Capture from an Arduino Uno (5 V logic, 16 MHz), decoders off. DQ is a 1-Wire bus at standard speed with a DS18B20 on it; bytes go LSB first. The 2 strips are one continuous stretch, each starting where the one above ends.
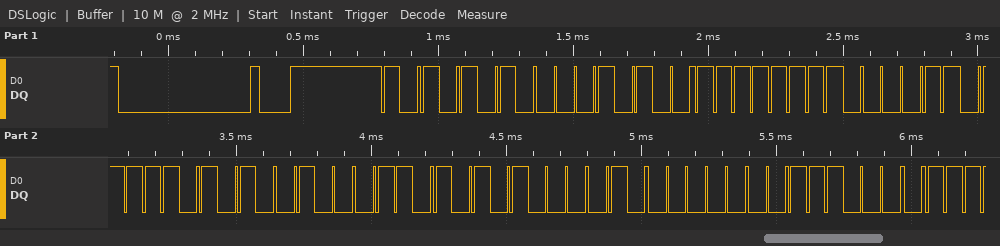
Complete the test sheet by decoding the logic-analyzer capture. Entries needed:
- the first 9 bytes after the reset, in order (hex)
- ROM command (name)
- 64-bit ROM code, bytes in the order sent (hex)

55 28 FF B0 57 62 15 02 1C
Match ROM
28 FF B0 57 62 15 02 1C
